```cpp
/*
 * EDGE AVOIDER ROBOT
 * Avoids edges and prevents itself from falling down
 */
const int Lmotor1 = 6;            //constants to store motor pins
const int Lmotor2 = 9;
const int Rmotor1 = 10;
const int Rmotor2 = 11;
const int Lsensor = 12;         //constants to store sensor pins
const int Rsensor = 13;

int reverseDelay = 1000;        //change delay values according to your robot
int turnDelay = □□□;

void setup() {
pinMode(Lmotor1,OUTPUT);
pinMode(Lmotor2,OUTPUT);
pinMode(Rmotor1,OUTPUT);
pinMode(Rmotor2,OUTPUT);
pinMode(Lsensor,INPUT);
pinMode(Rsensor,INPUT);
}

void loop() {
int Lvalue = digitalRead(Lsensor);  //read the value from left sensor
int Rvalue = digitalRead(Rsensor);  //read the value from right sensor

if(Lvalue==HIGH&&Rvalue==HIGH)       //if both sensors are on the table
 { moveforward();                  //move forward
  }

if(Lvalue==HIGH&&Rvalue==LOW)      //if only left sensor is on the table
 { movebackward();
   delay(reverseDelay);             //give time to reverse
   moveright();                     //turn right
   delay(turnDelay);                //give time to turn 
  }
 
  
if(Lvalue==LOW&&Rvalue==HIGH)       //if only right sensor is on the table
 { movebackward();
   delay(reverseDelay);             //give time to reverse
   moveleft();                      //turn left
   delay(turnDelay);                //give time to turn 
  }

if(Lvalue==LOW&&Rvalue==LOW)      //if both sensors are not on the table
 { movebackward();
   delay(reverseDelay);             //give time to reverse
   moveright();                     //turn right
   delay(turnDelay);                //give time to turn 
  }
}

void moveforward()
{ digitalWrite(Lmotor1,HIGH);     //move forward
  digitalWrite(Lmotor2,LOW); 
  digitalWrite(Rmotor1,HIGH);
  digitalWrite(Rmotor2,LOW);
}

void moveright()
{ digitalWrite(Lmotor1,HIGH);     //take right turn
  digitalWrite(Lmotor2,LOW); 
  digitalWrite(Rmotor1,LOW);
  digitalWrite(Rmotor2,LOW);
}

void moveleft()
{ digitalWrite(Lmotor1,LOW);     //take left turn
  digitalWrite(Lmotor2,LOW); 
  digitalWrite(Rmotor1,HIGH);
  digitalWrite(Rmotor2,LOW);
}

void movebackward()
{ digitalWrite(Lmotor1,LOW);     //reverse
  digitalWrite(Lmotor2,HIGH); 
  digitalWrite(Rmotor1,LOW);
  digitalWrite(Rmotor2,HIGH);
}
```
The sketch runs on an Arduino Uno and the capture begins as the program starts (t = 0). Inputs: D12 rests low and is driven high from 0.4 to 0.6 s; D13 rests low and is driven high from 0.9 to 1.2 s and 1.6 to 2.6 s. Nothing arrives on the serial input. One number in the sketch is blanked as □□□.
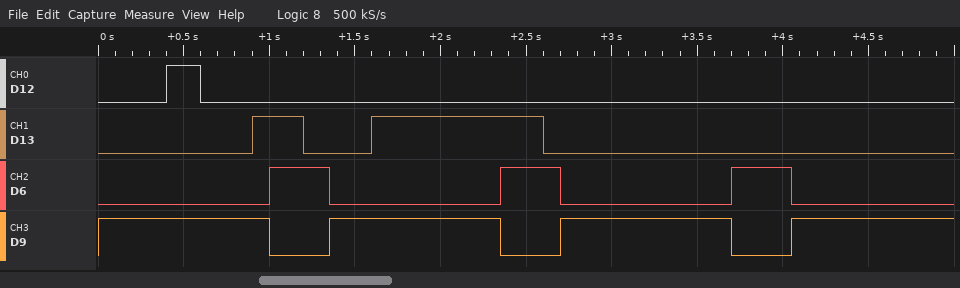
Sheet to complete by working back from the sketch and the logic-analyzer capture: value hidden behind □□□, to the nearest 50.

350
